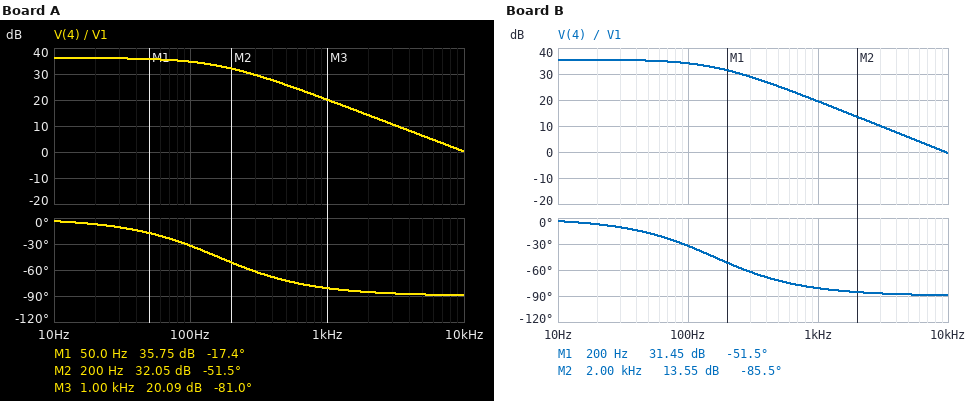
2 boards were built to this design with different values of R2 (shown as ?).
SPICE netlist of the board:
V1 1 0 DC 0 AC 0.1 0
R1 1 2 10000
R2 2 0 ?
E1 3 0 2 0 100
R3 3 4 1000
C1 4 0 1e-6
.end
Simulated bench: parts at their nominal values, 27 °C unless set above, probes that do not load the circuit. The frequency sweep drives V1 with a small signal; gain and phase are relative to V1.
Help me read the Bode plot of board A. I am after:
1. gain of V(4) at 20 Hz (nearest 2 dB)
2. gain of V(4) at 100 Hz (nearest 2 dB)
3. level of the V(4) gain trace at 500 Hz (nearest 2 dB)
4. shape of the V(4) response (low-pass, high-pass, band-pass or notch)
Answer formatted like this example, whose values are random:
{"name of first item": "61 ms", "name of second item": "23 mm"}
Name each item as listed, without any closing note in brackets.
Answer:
{"gain of V(4) at 20 Hz": "36 dB", "gain of V(4) at 100 Hz": "34 dB", "level of the V(4) gain trace at 500 Hz": "26 dB", "shape of the V(4) response": "low-pass"}
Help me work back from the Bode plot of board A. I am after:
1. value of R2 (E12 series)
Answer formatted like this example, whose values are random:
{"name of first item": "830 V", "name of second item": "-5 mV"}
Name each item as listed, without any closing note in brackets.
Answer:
{"value of R2": "18 kΩ"}
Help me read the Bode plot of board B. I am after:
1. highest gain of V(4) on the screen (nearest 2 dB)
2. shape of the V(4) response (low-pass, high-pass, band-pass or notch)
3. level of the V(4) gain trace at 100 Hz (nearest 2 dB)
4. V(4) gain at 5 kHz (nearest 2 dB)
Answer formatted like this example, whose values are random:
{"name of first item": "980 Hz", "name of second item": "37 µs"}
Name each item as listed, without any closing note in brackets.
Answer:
{"highest gain of V(4) on the screen": "36 dB", "shape of the V(4) response": "low-pass", "level of the V(4) gain trace at 100 Hz": "34 dB", "V(4) gain at 5 kHz": "6 dB"}
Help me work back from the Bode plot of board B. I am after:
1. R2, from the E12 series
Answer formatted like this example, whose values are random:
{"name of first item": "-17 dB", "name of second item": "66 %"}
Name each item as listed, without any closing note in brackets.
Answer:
{"R2, from the E12 series": "15 kΩ"}
